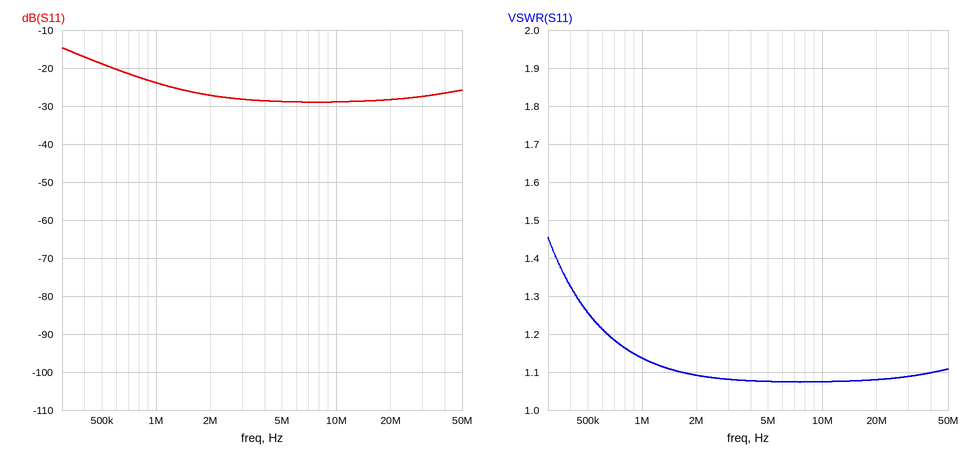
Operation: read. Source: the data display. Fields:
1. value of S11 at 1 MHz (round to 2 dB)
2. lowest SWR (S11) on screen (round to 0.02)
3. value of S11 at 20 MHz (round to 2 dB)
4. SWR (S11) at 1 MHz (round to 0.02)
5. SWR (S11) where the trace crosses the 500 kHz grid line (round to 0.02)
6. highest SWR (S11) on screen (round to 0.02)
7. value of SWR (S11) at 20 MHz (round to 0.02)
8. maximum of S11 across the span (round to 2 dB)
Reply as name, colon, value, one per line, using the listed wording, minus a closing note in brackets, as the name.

value of S11 at 1 MHz: -24 dB
lowest SWR (S11) on screen: 1.08
value of S11 at 20 MHz: -28 dB
SWR (S11) at 1 MHz: 1.14
SWR (S11) where the trace crosses the 500 kHz grid line: 1.26
highest SWR (S11) on screen: 1.46
value of SWR (S11) at 20 MHz: 1.08
maximum of S11 across the span: -14 dB
